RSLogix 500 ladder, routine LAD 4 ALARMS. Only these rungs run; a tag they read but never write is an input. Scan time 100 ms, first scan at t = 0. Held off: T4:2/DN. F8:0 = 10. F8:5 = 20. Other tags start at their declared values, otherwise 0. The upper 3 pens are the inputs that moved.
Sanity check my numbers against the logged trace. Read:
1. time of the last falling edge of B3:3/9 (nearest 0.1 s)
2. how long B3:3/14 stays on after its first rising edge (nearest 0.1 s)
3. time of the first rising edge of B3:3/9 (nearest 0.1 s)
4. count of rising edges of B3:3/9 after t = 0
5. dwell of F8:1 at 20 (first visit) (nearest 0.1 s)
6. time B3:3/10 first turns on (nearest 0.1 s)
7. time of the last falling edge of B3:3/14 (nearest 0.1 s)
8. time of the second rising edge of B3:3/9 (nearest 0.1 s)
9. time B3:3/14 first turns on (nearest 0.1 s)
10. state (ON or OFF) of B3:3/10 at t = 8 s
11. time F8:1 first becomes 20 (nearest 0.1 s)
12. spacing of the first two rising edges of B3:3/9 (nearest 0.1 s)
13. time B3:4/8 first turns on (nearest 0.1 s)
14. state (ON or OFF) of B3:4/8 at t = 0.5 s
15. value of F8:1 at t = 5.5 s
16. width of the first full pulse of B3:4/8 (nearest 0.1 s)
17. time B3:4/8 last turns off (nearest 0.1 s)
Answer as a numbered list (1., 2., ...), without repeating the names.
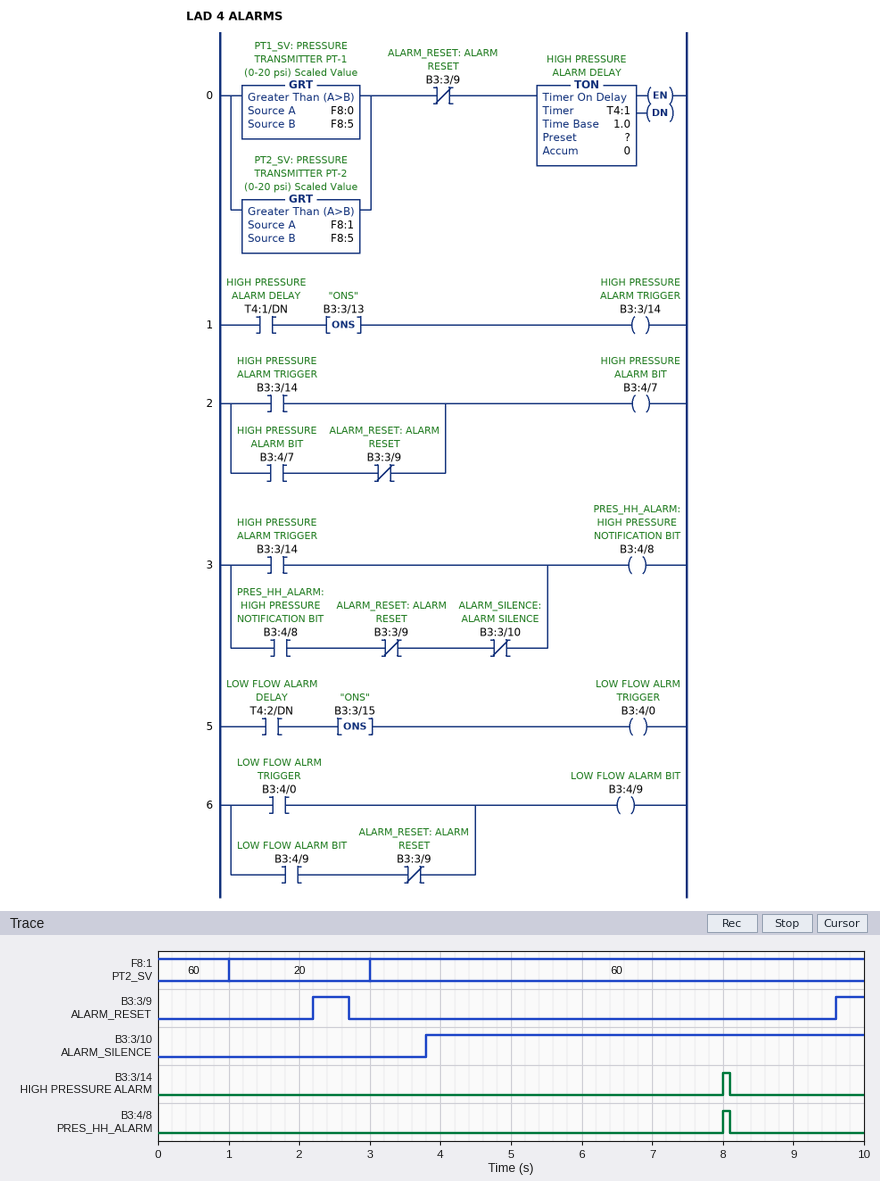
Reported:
1. 2.7 s
2. 0.1 s
3. 2.2 s
4. 2
5. 2.0 s
6. 3.8 s
7. 8.1 s
8. 9.6 s
9. 8.0 s
10. ON
11. 1.0 s
12. 7.4 s
13. 8.0 s
14. OFF
15. 60
16. 0.1 s
17. 8.1 s
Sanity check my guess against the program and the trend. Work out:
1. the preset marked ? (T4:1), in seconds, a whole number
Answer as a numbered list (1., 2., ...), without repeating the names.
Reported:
1. 5 s
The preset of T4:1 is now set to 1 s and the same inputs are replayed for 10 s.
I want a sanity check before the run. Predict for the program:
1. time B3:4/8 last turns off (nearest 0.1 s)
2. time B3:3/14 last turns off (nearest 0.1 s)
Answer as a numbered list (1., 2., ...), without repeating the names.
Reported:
1. 4.1 s
2. 4.1 s
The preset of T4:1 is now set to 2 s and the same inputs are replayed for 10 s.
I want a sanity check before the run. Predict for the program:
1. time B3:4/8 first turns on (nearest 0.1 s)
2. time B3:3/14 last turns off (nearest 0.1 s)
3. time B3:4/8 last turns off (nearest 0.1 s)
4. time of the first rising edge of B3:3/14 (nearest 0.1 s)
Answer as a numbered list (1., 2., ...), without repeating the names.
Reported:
1. 5.0 s
2. 5.1 s
3. 5.1 s
4. 5.0 s
